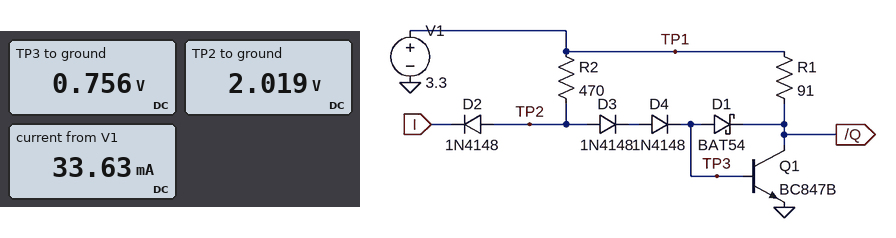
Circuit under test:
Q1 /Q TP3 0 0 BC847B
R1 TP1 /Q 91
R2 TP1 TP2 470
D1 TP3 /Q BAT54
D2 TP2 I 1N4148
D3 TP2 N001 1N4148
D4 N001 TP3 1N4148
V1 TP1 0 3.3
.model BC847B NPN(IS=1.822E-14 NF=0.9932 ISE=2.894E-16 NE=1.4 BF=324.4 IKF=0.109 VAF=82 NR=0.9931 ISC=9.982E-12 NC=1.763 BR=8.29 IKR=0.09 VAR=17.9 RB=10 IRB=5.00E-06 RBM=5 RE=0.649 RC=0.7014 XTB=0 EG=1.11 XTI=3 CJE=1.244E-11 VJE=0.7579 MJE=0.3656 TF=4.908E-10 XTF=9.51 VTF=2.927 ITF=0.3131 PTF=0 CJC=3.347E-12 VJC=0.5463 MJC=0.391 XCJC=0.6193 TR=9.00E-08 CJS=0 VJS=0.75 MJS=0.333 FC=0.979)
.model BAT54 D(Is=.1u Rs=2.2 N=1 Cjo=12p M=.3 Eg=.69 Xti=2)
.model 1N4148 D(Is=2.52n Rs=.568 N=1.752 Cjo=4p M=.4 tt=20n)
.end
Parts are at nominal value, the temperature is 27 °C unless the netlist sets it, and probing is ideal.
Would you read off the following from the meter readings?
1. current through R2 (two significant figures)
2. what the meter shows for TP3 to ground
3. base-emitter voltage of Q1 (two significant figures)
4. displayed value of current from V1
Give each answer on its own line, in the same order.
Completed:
2.7 mA
0.756 V
760 mV
33.63 mA
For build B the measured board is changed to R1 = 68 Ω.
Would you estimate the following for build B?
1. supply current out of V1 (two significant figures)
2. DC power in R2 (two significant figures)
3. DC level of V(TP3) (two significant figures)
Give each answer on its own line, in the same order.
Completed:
44 mA
3.4 mW
770 mV
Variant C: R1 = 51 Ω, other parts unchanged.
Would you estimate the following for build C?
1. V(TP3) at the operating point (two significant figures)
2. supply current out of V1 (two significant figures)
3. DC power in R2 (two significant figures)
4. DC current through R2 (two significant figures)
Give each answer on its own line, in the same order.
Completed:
790 mV
57 mA
3.3 mW
2.7 mA
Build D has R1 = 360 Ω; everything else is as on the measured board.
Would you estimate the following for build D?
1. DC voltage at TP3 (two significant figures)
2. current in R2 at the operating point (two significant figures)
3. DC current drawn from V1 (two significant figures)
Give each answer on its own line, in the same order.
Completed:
710 mV
2.8 mA
11 mA
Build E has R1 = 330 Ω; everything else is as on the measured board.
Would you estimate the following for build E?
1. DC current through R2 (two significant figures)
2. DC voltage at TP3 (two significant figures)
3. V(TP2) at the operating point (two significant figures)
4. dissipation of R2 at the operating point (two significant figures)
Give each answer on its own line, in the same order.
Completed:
2.8 mA
710 mV
2.0 V
3.7 mW
